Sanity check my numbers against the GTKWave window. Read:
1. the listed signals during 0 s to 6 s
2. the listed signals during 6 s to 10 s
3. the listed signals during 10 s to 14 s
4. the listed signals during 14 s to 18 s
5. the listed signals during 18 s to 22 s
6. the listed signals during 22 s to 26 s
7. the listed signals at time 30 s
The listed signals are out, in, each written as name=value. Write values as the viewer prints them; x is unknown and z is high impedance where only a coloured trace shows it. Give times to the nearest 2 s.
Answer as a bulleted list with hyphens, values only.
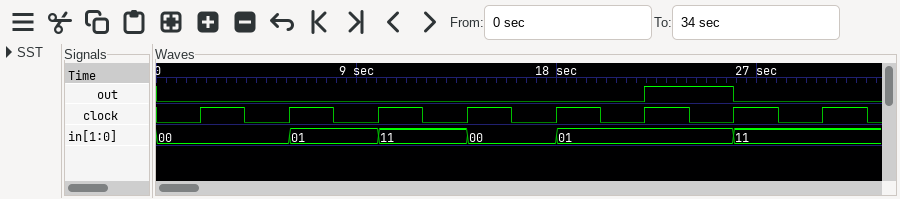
- out=0, in=00
- out=0, in=01
- out=0, in=11
- out=0, in=00
- out=0, in=01
- out=1, in=01
- out=0, in=11
